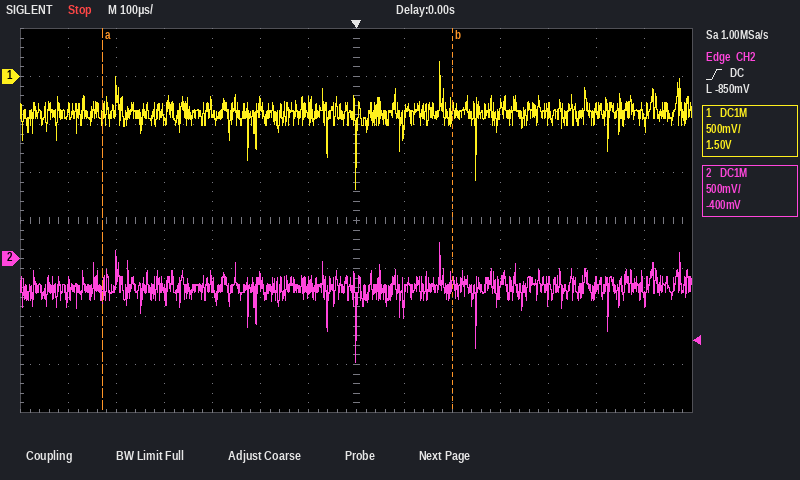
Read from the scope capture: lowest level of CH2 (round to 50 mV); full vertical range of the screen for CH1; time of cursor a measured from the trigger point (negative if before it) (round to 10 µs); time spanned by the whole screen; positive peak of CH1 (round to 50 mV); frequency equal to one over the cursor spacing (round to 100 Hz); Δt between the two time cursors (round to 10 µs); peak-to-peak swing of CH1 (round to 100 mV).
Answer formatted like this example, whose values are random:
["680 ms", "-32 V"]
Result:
["-1.10 V", "4 V", "-530 µs", "1.4 ms", "150 mV", "1.4 kHz", "730 µs", "1.30 V"]
